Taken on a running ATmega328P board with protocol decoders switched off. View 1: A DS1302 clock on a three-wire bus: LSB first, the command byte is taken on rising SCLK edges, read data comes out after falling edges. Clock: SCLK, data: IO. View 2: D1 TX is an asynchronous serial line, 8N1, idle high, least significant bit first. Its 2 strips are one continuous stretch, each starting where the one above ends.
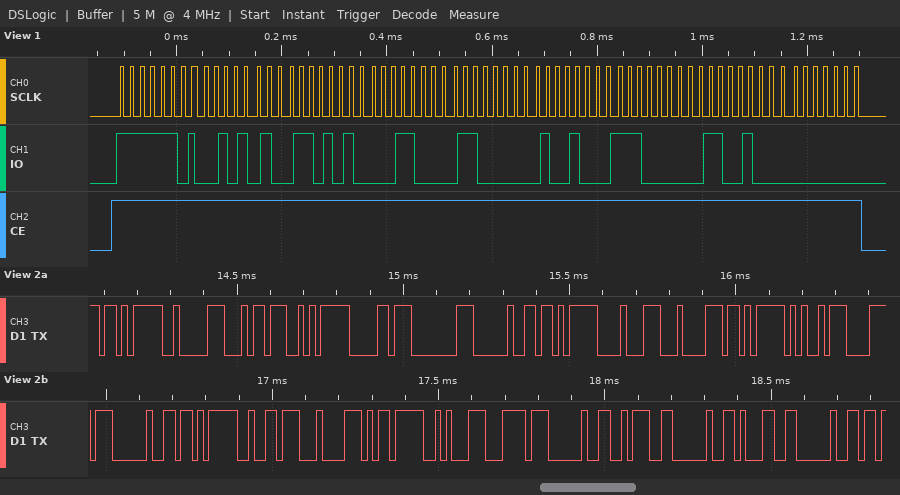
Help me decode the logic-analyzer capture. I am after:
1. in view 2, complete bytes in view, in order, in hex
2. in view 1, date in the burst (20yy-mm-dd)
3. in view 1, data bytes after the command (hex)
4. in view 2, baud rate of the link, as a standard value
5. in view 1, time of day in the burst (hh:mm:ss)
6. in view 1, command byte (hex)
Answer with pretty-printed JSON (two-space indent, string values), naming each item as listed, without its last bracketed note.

{
  "in view 2, complete bytes in view, in order, in hex": "EB 82 B4 EA B0 80 20 EB 88 84 EB A5 B8 20 EB B2 84 ED 8A BC 20 3A 20 31 20",
  "in view 1, date in the burst": "2026-12-06",
  "in view 1, data bytes after the command": "54 56 18 06 12 07 26 00",
  "in view 2, baud rate of the link, as a standard value": "57600 baud",
  "in view 1, time of day in the burst": "18:56:54",
  "in view 1, command byte": "0xBF"
}
